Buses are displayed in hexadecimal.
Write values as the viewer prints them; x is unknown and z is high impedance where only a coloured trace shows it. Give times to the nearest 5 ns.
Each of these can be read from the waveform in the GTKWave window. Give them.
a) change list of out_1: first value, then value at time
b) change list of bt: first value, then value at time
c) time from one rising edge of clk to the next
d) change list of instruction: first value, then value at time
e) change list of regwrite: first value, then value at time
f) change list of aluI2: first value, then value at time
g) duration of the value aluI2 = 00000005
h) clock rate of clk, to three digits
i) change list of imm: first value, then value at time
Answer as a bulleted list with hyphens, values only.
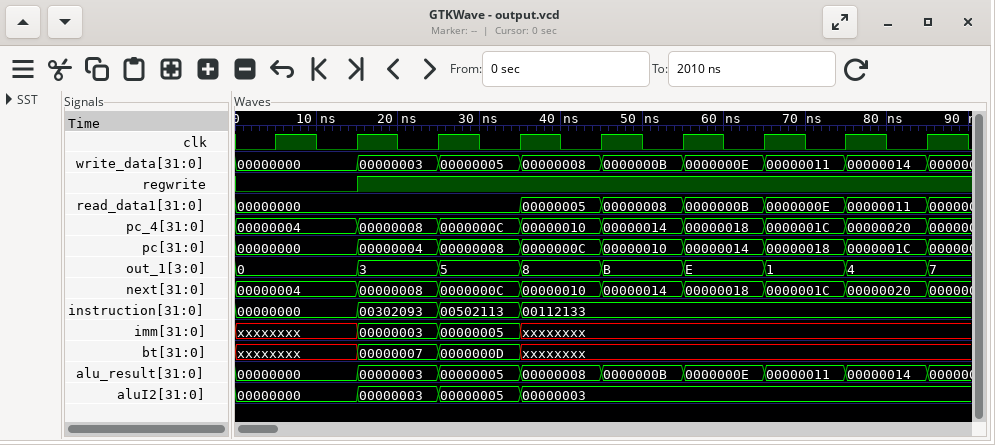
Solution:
- 0, 3 at 15 ns, 5 at 25 ns, 8 at 35 ns, B at 45 ns, E at 55 ns, 1 at 65 ns, 4 at 75 ns, 7 at 85 ns
- xxxxxxxx, 00000007 at 15 ns, 0000000D at 25 ns, xxxxxxxx at 35 ns
- 10 ns
- 00000000, 00302093 at 15 ns, 00502113 at 25 ns, 00112133 at 35 ns
- 0, 1 at 15 ns
- 00000000, 00000003 at 15 ns, 00000005 at 25 ns, 00000003 at 35 ns
- 10 ns
- 100 MHz
- xxxxxxxx, 00000003 at 15 ns, 00000005 at 25 ns, xxxxxxxx at 35 ns
